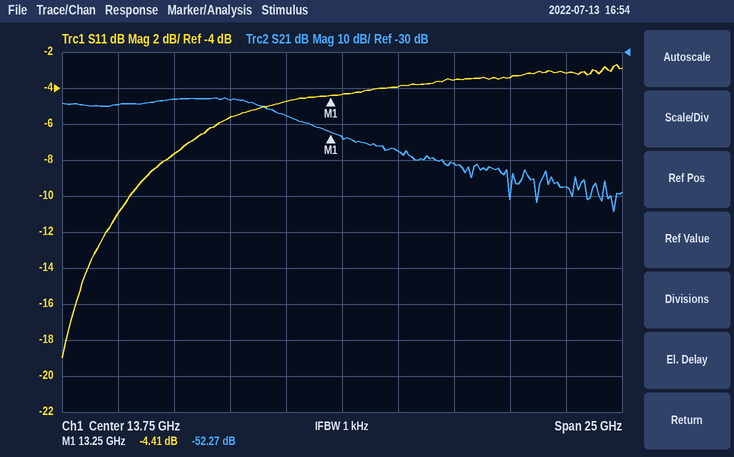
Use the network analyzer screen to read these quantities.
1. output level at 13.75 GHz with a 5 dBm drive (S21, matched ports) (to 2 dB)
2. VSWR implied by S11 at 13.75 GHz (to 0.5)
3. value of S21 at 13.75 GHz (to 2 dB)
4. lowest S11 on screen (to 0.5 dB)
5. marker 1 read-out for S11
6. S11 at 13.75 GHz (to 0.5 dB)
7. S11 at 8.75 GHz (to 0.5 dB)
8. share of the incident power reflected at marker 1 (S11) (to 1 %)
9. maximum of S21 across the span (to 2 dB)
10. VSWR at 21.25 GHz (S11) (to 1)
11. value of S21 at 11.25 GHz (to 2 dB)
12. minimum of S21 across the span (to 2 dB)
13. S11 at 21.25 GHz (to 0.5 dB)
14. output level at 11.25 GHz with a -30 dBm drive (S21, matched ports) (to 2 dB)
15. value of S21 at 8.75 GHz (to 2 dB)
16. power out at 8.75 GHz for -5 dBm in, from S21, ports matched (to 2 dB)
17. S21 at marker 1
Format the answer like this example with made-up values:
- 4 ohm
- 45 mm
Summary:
- -48 dBm
- 4.0
- -54 dB
- -19.0 dB
- -4.41 dB
- -4.5 dB
- -5.5 dB
- 36 %
- -42 dB
- 5
- -48 dB
- -74 dB
- -3.5 dB
- -78 dBm
- -44 dB
- -48 dBm
- -52.27 dB
